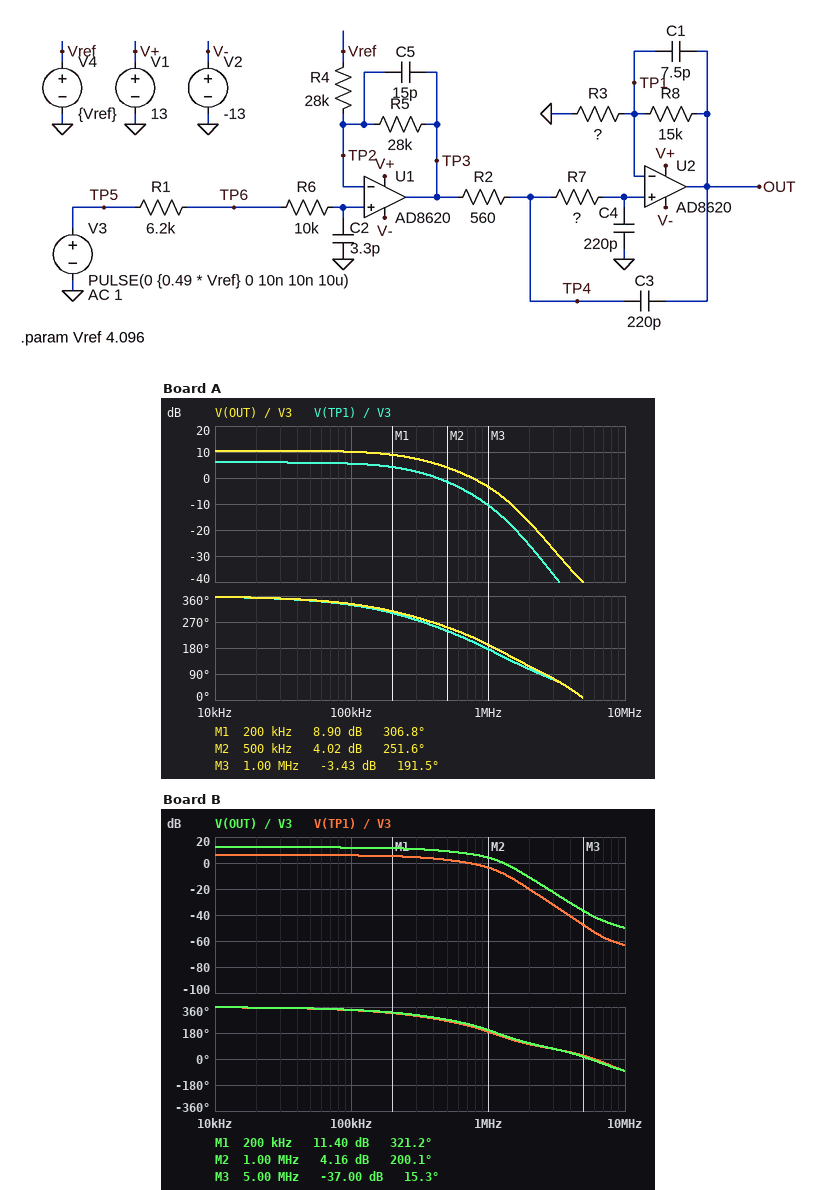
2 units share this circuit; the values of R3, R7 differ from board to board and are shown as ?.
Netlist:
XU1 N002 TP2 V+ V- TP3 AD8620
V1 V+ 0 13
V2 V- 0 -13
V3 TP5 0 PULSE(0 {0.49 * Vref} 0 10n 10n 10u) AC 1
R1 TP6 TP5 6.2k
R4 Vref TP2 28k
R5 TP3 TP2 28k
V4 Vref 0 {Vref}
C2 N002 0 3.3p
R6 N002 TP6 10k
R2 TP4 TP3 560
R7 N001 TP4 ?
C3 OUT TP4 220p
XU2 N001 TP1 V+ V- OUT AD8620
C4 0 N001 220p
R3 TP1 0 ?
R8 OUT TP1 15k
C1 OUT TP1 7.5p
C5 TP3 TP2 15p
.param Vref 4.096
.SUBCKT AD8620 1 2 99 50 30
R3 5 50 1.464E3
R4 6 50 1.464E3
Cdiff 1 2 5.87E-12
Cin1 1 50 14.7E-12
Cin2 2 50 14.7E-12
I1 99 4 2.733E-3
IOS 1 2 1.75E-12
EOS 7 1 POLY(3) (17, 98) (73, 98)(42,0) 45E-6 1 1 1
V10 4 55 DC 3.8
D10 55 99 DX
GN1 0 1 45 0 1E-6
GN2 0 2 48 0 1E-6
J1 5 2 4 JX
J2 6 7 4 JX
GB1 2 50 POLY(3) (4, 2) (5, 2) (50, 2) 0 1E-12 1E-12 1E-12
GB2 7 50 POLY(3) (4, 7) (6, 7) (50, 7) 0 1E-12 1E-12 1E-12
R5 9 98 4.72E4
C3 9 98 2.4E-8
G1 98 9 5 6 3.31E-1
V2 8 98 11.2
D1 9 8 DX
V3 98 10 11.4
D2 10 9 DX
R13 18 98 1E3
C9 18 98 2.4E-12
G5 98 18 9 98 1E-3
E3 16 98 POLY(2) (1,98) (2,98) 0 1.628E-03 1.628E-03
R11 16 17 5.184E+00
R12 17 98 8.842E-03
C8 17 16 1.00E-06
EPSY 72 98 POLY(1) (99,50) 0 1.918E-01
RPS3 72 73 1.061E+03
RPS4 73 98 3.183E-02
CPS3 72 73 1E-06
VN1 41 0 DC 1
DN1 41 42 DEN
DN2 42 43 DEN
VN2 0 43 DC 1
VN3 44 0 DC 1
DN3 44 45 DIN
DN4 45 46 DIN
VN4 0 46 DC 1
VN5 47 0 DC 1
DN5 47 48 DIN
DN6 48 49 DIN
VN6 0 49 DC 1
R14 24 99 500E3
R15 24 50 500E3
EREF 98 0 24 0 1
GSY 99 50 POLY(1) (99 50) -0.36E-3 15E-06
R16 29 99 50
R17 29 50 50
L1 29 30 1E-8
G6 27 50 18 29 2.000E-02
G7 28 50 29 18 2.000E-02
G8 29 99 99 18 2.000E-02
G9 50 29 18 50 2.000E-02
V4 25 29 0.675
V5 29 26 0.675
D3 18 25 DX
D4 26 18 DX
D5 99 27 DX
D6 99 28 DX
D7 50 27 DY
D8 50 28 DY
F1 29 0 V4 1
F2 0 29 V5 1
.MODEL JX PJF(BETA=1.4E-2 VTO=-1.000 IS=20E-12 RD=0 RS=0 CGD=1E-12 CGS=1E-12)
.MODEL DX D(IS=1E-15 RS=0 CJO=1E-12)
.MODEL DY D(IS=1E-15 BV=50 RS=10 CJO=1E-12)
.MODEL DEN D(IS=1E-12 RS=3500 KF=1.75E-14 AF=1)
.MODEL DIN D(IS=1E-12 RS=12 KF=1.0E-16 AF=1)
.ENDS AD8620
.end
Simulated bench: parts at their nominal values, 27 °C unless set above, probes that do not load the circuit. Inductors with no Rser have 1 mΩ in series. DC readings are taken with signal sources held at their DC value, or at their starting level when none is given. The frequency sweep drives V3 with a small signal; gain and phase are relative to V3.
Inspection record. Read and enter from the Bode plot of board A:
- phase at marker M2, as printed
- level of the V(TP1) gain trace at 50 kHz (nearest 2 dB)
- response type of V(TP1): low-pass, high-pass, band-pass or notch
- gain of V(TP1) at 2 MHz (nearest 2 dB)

251.6 deg
6 dB
low-pass
-26 dB
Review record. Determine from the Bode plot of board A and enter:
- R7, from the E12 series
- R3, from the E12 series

2.2 kΩ
22 kΩ
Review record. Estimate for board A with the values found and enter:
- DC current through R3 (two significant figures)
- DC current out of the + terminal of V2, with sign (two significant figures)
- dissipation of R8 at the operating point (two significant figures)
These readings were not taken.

190 µA
-5.9 mA
520 µW
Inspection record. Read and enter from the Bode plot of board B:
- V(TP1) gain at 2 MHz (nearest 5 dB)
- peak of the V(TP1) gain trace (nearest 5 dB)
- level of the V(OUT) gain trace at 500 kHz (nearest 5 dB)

-20 dB
5 dB
10 dB
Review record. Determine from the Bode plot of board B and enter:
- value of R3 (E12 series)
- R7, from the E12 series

15 kΩ
1.2 kΩ
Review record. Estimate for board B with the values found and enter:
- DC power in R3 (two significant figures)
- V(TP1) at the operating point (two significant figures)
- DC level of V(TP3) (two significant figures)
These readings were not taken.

1.1 mW
-4.1 V
-4.1 V
